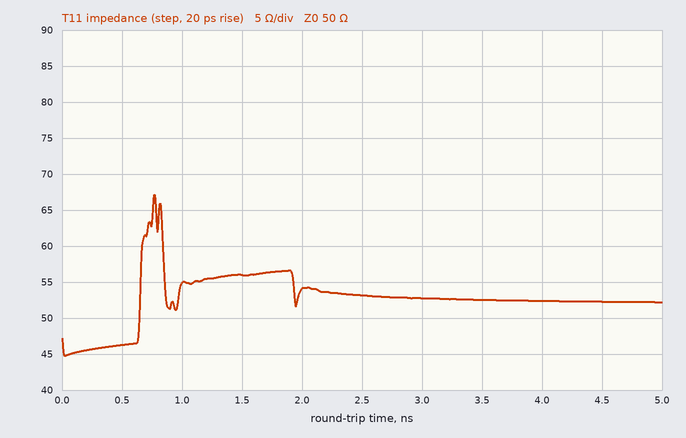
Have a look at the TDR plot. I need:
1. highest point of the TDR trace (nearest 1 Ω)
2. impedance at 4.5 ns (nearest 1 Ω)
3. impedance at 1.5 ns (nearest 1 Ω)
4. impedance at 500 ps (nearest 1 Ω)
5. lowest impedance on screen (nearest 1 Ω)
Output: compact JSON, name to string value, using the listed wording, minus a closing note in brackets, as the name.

{"highest point of the TDR trace": "67 Ω", "impedance at 4.5 ns": "52 Ω", "impedance at 1.5 ns": "56 Ω", "impedance at 500 ps": "46 Ω", "lowest impedance on screen": "45 Ω"}
